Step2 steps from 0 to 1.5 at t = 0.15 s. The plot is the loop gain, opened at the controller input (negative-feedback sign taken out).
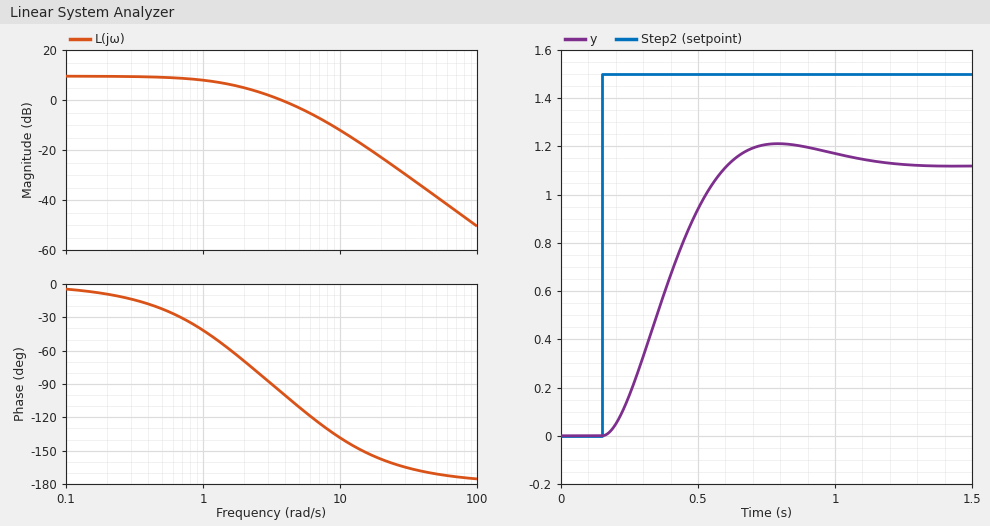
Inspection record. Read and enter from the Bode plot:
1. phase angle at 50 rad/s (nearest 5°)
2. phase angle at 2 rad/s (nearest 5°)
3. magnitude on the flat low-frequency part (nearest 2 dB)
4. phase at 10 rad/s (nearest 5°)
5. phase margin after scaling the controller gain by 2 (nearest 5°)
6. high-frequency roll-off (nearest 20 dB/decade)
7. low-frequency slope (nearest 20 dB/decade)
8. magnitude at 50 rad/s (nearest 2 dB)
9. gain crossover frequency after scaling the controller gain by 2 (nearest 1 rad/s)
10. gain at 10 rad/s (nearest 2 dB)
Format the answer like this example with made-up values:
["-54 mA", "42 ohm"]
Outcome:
["-170°", "-70°", "10 dB", "-140°", "60°", "-40 dB/decade", "0 dB/decade", "-38 dB", "6 rad/s", "-12 dB"]
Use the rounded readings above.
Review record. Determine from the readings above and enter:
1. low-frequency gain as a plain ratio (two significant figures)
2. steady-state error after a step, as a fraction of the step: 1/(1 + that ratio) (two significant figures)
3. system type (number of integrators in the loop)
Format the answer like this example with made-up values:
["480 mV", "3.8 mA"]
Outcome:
["3.2", "0.24", "0"]
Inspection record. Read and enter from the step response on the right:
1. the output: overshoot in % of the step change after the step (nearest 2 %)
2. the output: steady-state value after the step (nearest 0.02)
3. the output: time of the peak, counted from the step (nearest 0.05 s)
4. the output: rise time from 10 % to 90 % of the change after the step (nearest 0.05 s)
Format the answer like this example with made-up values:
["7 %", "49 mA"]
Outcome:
["8 %", "1.12", "0.65 s", "0.30 s"]
